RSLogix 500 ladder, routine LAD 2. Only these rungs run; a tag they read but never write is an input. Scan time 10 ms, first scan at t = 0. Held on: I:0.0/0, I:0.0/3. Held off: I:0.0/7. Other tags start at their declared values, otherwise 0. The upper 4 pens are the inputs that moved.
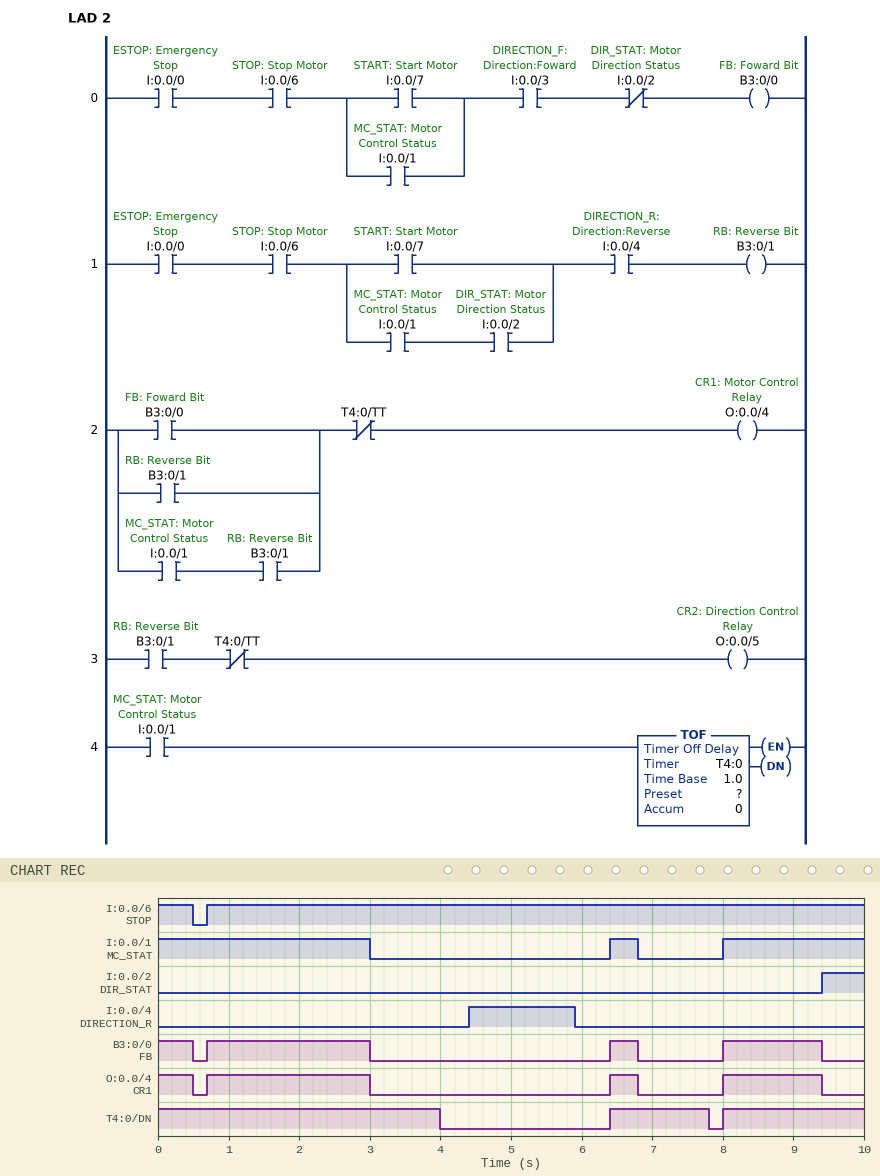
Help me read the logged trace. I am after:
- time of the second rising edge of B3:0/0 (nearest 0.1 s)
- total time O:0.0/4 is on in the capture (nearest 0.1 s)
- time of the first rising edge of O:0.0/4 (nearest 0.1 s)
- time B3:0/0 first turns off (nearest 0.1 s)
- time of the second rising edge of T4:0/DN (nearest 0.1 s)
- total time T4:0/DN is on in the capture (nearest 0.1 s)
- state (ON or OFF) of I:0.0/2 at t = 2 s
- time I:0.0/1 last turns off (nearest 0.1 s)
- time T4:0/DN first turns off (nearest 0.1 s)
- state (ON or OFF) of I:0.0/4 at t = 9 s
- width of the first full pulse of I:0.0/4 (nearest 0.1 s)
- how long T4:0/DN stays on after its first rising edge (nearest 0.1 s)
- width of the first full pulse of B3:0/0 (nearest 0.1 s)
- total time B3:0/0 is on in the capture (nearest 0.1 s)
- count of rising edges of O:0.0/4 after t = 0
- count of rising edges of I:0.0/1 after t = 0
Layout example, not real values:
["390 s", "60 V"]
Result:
["6.4 s", "4.6 s", "0.7 s", "0.5 s", "8.0 s", "7.4 s", "OFF", "6.8 s", "4.0 s", "OFF", "1.5 s", "1.4 s", "2.3 s", "4.6 s", "3", "2"]
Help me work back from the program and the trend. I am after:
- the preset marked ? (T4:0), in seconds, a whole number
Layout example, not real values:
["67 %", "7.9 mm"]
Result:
["1 s"]
